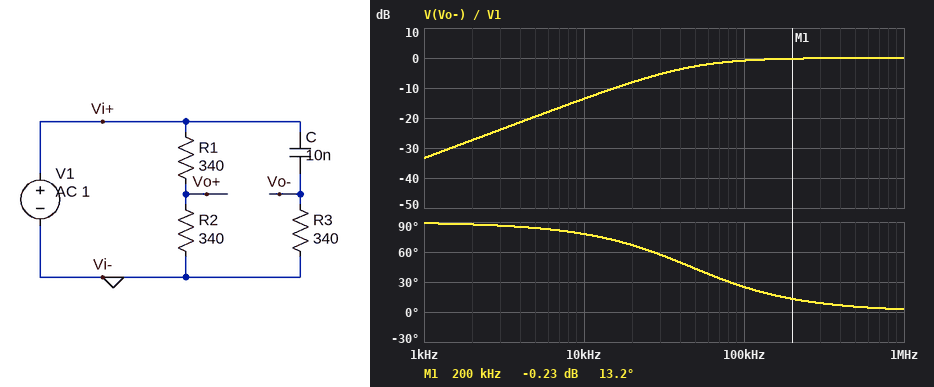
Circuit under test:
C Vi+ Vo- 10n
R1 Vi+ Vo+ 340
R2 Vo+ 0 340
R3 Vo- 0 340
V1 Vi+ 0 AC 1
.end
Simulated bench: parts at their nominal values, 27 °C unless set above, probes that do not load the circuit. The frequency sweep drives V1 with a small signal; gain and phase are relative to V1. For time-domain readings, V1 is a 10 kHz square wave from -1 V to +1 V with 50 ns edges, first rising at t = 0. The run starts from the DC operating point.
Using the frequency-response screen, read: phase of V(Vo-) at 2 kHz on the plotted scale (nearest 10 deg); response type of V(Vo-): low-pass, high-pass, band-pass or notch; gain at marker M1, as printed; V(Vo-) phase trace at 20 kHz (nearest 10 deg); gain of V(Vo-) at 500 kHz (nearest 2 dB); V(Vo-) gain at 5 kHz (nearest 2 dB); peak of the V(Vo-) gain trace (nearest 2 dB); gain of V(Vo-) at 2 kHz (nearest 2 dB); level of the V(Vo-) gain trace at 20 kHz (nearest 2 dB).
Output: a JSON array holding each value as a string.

["90 deg", "high-pass", "-0.23 dB", "70 deg", "0 dB", "-20 dB", "0 dB", "-28 dB", "-8 dB"]
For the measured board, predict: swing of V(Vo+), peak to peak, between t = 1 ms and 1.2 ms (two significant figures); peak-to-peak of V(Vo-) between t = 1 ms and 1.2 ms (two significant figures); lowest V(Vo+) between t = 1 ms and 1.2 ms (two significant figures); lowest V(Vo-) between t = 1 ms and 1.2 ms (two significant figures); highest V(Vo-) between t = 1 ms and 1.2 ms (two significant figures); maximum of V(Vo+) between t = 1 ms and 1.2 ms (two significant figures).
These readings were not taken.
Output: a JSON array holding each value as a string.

["1.0 V", "4.0 V", "-500 mV", "-2.0 V", "2.0 V", "500 mV"]
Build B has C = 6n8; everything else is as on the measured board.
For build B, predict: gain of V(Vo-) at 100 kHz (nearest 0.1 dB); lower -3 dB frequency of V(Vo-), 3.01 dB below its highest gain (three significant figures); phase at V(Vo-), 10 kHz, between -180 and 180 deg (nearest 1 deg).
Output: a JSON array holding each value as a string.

["-1.7 dB", "68.8 kHz", "82 deg"]
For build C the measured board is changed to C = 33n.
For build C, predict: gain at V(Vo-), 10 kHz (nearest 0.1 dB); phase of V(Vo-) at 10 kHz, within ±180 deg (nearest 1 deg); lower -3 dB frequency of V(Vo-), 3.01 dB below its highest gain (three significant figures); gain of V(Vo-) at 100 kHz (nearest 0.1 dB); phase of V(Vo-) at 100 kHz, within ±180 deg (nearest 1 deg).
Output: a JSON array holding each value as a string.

["-4.8 dB", "55 deg", "14.2 kHz", "-0.1 dB", "8 deg"]
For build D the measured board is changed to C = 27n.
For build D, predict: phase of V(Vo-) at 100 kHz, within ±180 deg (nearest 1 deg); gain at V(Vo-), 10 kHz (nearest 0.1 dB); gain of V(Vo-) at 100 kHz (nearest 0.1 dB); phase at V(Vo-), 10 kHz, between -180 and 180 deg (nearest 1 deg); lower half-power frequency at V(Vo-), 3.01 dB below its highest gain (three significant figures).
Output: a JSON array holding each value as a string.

["10 deg", "-6.0 dB", "-0.1 dB", "60 deg", "17.3 kHz"]
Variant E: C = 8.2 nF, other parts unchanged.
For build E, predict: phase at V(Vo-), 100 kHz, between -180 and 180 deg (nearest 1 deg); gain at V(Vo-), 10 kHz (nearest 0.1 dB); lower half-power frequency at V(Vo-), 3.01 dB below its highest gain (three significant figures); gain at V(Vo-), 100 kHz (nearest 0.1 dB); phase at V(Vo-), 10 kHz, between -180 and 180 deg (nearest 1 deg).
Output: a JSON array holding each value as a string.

["30 deg", "-15.3 dB", "57.1 kHz", "-1.2 dB", "80 deg"]
